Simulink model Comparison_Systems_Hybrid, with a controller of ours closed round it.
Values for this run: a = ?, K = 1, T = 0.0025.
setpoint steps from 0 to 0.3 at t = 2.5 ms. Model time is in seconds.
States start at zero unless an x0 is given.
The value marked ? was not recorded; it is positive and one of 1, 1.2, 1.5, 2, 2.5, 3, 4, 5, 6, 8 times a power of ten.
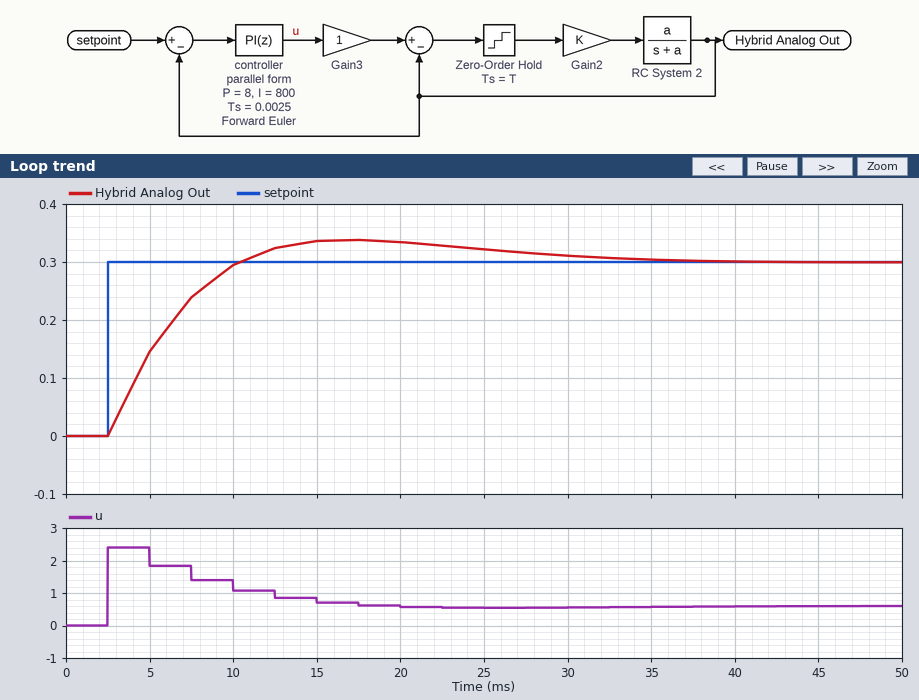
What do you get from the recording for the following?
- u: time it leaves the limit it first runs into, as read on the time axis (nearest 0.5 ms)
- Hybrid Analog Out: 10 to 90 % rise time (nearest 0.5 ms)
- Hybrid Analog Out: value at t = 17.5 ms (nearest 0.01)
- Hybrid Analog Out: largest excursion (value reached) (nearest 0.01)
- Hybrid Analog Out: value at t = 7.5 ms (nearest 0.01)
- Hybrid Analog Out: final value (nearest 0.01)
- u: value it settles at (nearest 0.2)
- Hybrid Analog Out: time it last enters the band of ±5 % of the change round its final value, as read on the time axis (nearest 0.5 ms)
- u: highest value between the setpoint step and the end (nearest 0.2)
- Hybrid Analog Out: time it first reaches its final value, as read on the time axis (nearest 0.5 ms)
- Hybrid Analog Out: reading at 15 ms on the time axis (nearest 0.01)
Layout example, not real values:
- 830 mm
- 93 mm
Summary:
- 5.0 ms
- 6.0 ms
- 0.34
- 0.34
- 0.24
- 0.30
- 0.6
- 28.0 ms
- 2.4
- 10.5 ms
- 0.34
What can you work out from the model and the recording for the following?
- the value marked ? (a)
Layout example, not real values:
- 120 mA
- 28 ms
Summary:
- 25
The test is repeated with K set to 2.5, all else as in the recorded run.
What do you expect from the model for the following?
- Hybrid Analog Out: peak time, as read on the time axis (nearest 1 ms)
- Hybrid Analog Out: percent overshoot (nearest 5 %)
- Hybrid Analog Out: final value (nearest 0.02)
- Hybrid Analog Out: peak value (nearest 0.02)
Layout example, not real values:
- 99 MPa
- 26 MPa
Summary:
- 5 ms
- 20 %
- 0.30
- 0.36
